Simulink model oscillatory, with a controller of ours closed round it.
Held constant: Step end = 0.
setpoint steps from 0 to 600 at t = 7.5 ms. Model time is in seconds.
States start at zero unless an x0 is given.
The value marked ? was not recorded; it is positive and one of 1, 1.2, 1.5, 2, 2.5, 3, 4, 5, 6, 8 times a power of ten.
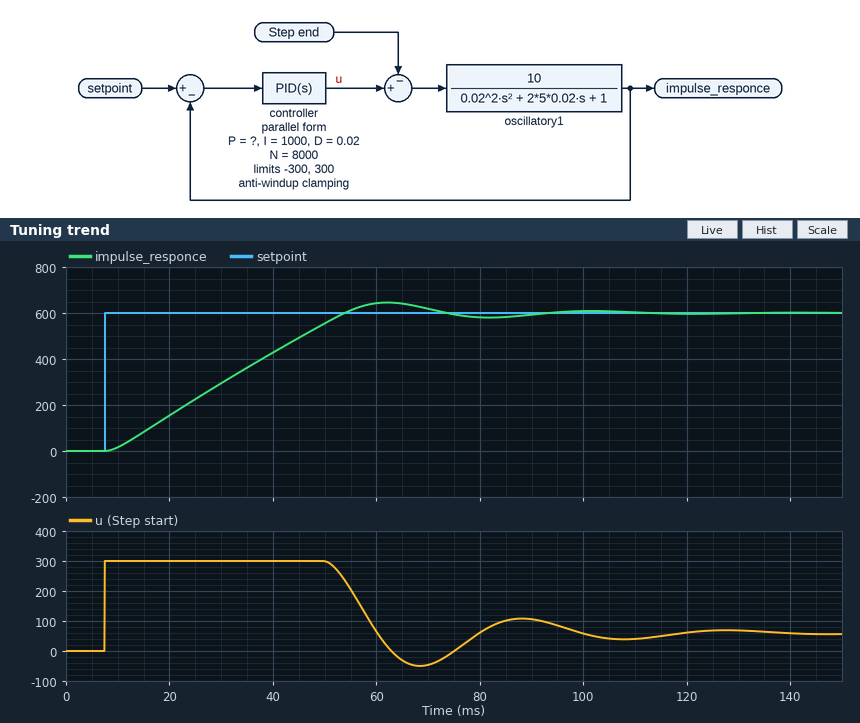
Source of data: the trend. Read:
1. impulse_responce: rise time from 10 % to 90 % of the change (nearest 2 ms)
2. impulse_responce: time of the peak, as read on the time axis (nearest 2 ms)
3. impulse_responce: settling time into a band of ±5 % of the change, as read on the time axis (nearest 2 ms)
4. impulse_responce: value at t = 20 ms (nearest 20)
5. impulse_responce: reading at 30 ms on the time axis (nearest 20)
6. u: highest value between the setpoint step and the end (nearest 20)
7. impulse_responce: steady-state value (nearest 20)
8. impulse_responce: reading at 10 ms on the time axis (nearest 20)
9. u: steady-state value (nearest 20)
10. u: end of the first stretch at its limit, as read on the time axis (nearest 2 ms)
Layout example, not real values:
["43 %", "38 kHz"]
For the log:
["36 ms", "62 ms", "68 ms", "160", "300", "300", "600", "20", "60", "50 ms"]
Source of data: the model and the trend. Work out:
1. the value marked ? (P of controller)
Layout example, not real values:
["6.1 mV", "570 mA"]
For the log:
["4"]
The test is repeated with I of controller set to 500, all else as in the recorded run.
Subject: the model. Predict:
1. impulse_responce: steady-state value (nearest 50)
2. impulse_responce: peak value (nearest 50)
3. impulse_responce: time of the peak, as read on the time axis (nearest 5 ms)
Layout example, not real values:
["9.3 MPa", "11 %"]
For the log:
["600", "650", "65 ms"]
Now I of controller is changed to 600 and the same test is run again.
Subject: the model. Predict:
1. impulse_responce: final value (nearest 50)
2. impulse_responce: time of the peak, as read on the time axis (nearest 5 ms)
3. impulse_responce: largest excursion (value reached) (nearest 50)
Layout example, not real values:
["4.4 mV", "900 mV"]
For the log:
["600", "65 ms", "650"]
